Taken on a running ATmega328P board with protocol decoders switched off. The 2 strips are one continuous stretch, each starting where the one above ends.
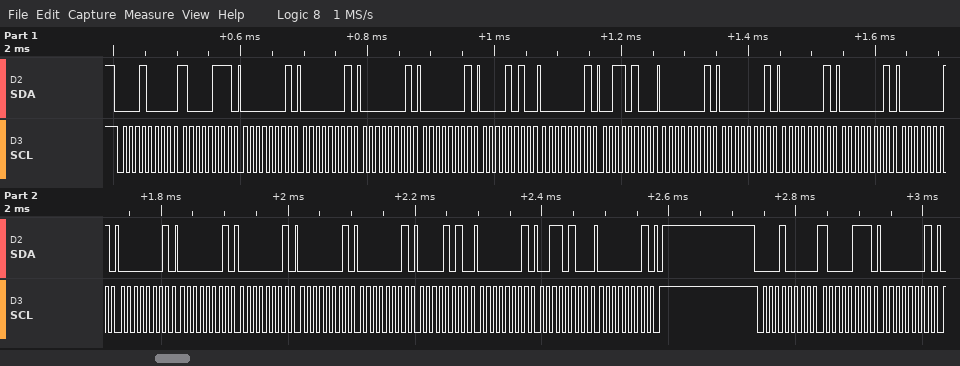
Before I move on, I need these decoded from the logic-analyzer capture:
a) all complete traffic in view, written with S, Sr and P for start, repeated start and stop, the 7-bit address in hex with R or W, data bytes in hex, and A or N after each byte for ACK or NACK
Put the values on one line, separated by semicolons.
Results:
S 08W A 87 A 01 A 01 A 01 A 01 A 0A A 01 A 34 A 01 A 01 A 01 A 01 A 01 A 01 A 01 A 01 A 01 A 01 A 0A A 01 A 34 A 01 A P S 08W A 87 A 01 A
